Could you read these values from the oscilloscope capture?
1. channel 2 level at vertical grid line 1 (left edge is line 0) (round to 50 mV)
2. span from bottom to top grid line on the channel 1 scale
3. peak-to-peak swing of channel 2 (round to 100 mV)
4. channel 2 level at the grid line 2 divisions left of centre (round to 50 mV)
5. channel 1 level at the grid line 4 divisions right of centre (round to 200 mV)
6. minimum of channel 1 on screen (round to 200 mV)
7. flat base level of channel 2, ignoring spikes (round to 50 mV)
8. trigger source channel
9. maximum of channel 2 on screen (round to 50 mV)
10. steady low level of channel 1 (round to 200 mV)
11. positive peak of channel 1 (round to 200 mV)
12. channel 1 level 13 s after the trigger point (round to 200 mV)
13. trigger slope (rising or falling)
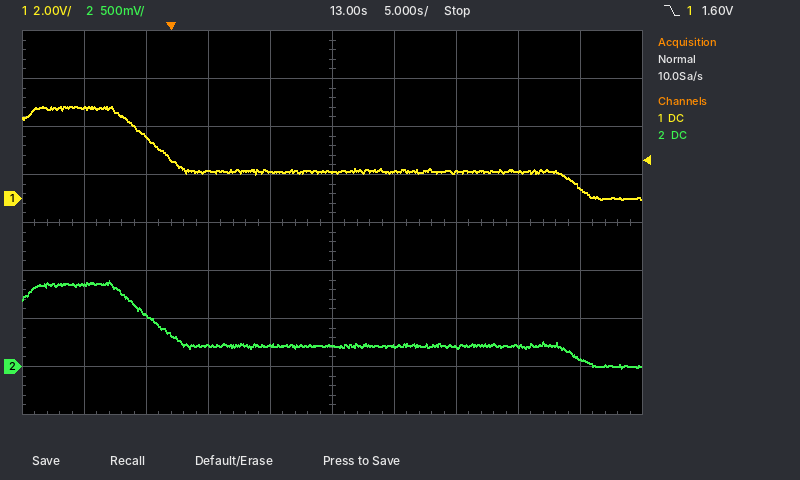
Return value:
850 mV
16 V
900 mV
200 mV
400 mV
0.0 V
200 mV
channel 1
900 mV
1.2 V
3.8 V
1.2 V
falling
